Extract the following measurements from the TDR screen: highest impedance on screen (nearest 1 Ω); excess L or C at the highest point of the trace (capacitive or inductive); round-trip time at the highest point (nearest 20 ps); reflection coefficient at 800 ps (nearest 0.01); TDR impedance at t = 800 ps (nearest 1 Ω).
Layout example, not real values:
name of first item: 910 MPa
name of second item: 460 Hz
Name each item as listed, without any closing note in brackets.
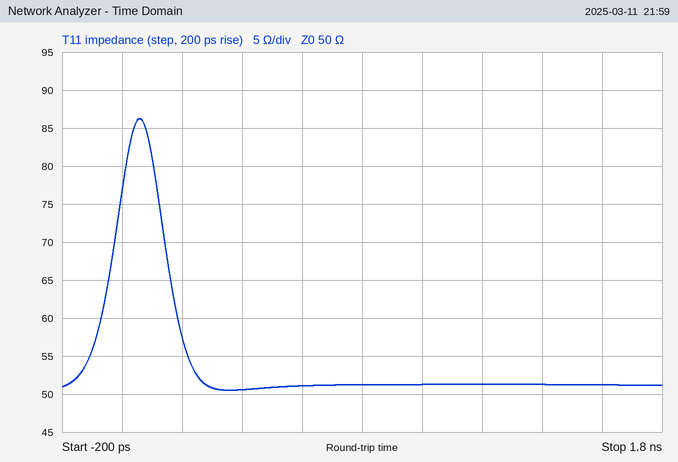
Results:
highest impedance on screen: 86 Ω
excess L or C at the highest point of the trace: inductive
round-trip time at the highest point: 60 ps
reflection coefficient at 800 ps: +0.01
TDR impedance at t = 800 ps: 51 Ω
